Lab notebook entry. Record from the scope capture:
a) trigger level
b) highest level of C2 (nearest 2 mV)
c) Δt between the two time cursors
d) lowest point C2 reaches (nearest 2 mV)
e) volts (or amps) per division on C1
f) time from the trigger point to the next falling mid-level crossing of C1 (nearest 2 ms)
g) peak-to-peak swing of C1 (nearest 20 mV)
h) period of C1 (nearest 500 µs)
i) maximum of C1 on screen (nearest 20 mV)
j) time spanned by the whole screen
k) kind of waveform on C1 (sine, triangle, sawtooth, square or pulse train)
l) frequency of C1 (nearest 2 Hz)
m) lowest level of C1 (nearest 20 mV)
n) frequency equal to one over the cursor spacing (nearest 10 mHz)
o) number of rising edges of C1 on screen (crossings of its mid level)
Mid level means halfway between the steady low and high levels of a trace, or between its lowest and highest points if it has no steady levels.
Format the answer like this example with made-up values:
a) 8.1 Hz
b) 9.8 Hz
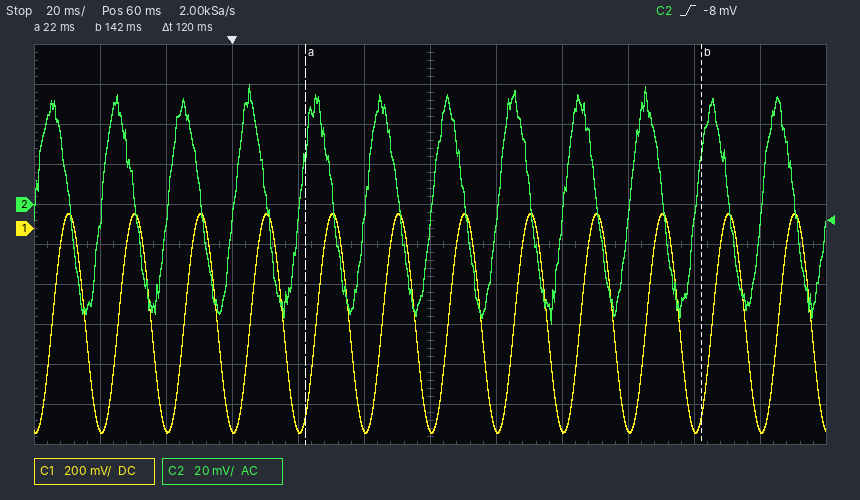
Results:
a) -8 mV
b) 60 mV
c) 120 ms
d) -60 mV
e) 200 mV
f) 16 ms
g) 1.10 V
h) 20.0 ms
i) 80 mV
j) 240 ms
k) sine
l) 50 Hz
m) -1.02 V
n) 8.33 Hz
o) 12
